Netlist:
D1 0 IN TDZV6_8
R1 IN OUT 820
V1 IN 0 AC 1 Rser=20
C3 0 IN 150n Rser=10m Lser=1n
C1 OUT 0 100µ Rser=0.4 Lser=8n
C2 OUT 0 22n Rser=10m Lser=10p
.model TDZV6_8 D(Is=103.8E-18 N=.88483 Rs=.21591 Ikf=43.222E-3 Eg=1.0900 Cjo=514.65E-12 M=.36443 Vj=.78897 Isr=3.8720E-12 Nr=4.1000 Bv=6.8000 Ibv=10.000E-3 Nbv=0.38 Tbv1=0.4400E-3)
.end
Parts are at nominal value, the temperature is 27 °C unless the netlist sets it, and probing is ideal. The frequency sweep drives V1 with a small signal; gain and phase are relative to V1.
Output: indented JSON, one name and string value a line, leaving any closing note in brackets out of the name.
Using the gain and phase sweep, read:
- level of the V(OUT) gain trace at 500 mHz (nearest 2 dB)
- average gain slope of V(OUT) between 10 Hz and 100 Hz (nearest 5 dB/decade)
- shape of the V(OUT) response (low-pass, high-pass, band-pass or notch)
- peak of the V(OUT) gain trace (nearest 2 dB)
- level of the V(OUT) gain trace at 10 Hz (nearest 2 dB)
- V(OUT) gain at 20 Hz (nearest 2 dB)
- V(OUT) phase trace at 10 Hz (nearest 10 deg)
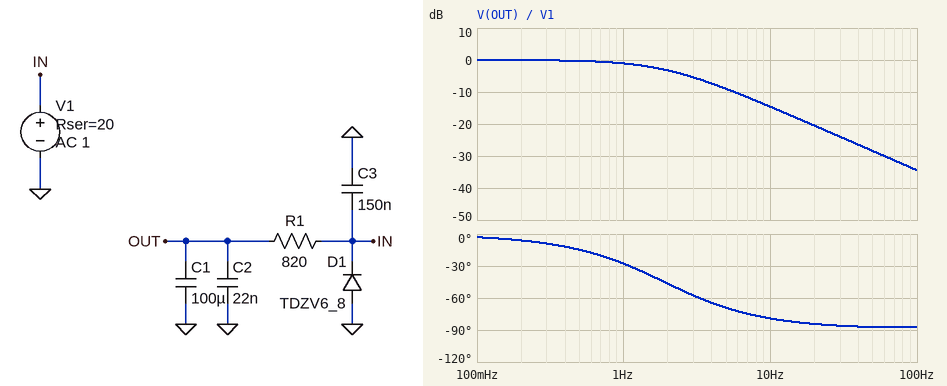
{
  "level of the V(OUT) gain trace at 500 mHz": "0 dB",
  "average gain slope of V(OUT) between 10 Hz and 100 Hz": "-20 dB/decade",
  "shape of the V(OUT) response": "low-pass",
  "peak of the V(OUT) gain trace": "0 dB",
  "level of the V(OUT) gain trace at 10 Hz": "-14 dB",
  "V(OUT) gain at 20 Hz": "-20 dB",
  "V(OUT) phase trace at 10 Hz": "-80 deg"
}
